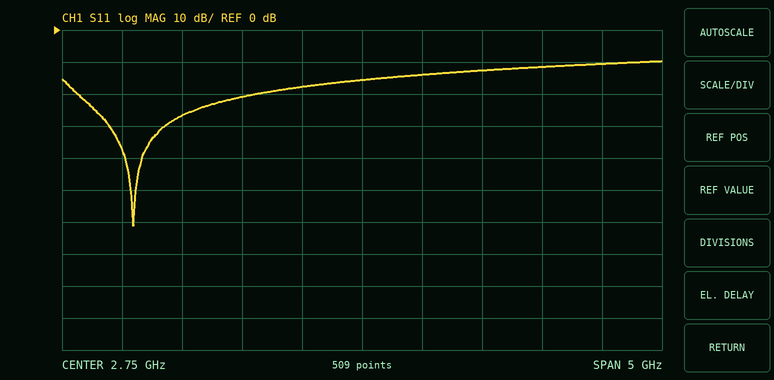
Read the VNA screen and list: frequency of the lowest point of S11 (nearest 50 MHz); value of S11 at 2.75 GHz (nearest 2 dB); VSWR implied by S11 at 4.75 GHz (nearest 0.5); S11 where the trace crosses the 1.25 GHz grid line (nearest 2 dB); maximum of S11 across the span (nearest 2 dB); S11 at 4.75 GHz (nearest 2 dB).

850 MHz
-16 dB
2.0
-26 dB
-10 dB
-10 dB
